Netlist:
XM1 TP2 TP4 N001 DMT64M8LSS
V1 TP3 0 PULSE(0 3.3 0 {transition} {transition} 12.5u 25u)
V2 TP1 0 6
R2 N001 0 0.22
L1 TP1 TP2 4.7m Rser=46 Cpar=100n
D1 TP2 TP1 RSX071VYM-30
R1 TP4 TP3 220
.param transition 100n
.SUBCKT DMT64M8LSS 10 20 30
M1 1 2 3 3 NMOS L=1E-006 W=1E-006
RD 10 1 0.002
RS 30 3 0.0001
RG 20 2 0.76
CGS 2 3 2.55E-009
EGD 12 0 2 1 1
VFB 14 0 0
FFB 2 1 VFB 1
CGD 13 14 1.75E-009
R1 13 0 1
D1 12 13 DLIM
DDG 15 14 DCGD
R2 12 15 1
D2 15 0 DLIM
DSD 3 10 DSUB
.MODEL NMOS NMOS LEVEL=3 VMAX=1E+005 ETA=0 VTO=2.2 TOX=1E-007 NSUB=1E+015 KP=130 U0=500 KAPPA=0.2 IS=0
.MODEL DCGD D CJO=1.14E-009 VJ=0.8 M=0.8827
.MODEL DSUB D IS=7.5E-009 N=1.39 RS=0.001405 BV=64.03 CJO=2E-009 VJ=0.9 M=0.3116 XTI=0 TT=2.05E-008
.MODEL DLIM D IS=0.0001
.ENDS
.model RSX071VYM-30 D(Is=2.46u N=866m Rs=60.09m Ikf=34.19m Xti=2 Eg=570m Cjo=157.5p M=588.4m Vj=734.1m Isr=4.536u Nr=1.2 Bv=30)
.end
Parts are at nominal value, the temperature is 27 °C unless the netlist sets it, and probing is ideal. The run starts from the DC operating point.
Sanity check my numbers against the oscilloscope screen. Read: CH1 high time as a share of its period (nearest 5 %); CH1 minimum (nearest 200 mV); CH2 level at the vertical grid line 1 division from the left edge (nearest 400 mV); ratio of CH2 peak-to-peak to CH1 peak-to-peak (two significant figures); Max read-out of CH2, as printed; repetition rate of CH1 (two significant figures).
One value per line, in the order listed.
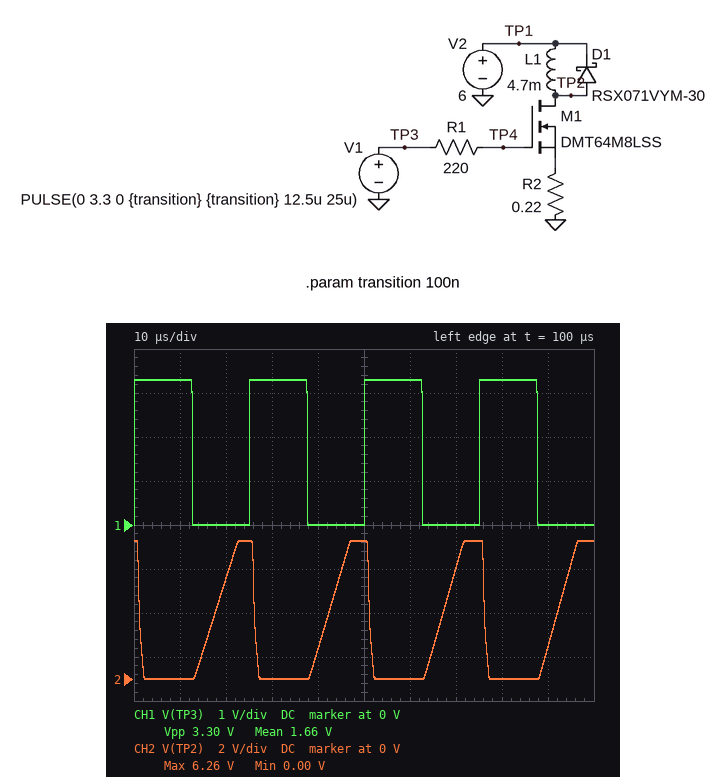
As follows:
50 %
0 V
0 V
1.9
6.26 V
40 kHz
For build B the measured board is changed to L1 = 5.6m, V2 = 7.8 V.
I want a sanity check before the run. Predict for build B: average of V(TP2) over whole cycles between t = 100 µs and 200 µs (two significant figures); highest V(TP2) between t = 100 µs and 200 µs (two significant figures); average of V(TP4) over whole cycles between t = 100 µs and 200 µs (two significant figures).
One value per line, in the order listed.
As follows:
2.7 V
8.1 V
1.7 V
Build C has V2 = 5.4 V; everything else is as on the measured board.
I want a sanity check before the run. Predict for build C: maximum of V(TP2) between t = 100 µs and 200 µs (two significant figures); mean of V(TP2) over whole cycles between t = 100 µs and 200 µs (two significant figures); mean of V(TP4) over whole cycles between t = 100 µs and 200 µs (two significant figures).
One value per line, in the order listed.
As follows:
5.7 V
2.0 V
1.7 V
